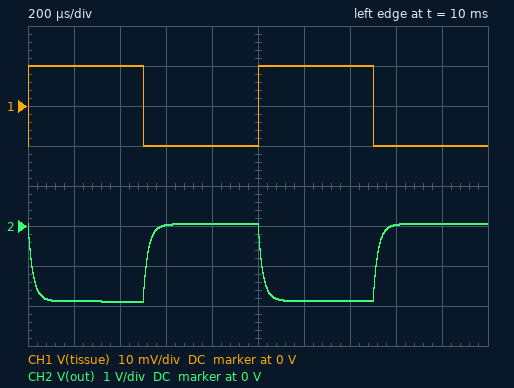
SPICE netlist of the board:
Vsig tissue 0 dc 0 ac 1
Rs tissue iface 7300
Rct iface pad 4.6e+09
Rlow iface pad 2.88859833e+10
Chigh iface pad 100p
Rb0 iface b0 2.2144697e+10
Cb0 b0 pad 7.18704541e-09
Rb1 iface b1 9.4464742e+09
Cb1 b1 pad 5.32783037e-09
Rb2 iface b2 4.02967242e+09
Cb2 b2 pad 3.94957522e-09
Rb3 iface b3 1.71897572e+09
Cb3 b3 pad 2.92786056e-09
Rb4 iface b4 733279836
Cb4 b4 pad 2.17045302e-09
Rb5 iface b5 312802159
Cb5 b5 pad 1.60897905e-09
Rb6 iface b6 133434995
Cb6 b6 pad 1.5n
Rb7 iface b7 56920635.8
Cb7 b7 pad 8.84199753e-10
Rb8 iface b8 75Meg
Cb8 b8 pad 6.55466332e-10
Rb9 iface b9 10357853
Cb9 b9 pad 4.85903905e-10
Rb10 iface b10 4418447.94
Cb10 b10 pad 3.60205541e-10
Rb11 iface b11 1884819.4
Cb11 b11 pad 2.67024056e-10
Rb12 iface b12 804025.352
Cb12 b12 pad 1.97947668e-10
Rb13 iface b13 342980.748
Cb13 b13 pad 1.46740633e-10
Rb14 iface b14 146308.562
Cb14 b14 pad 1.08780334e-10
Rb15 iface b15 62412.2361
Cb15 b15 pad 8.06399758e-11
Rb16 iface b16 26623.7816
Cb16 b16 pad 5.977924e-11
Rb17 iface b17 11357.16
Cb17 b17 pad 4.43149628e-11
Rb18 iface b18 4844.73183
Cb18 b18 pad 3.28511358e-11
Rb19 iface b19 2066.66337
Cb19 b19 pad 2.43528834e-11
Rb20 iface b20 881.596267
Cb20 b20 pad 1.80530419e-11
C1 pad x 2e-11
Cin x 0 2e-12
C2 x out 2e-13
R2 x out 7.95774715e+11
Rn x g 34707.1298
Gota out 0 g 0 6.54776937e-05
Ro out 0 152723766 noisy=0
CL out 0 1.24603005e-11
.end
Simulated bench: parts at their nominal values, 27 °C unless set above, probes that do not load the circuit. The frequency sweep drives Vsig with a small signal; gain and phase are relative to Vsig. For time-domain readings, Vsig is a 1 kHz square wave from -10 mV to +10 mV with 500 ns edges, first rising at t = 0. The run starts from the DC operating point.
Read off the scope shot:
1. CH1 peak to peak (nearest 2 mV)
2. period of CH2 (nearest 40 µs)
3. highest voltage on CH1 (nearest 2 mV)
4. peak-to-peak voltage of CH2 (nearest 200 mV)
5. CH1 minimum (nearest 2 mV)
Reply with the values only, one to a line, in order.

20 mV
1.00 ms
10 mV
2.0 V
-10 mV
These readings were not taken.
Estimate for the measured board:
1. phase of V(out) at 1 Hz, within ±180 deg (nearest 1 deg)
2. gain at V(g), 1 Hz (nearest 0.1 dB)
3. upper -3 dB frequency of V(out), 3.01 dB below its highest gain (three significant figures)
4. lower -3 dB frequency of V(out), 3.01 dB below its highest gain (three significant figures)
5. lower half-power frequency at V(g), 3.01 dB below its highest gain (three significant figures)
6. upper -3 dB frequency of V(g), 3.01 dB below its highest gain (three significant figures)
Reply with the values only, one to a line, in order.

-135 deg
-43.1 dB
7.20 kHz
976 mHz
7.71 kHz
11.1 MHz
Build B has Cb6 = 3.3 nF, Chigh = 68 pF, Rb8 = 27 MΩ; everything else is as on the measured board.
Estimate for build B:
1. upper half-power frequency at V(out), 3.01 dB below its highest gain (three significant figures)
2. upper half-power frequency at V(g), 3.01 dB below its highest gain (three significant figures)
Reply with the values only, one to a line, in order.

7.16 kHz
11.0 MHz
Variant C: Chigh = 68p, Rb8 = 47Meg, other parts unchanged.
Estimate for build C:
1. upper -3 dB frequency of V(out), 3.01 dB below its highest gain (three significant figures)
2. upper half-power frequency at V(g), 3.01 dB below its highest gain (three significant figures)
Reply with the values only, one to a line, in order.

7.17 kHz
11.0 MHz
